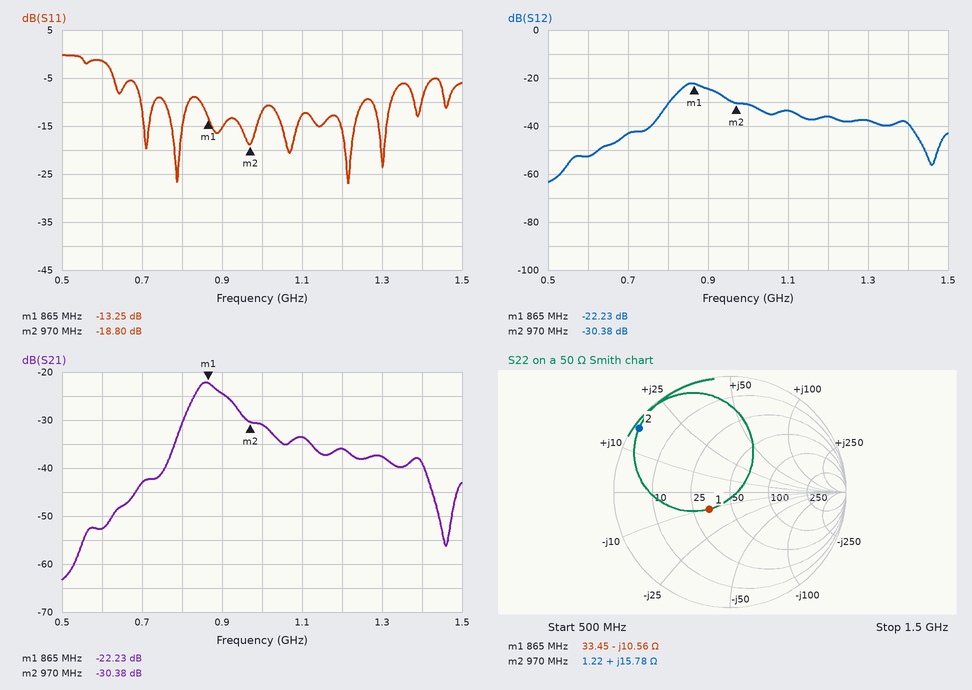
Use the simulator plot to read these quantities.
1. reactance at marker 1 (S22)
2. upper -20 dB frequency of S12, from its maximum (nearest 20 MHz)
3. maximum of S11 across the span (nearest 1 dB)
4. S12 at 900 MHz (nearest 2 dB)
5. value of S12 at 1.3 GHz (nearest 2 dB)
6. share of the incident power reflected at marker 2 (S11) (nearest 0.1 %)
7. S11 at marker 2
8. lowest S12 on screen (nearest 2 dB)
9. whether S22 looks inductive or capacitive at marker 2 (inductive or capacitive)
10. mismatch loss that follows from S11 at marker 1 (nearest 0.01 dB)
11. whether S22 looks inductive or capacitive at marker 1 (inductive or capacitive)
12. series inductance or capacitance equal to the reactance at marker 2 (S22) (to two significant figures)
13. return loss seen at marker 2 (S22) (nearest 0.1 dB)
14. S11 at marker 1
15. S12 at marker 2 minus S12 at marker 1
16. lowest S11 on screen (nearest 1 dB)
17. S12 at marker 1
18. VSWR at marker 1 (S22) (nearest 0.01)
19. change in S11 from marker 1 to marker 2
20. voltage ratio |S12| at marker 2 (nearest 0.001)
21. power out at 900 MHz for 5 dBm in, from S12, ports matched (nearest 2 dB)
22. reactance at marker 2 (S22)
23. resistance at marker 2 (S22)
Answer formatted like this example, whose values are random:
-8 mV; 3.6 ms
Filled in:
-10.56 Ω; 1.42 GHz; 0 dB; -24 dB; -38 dB; 1.3 %; -18.80 dB; -64 dB; inductive; 0.21 dB; capacitive; 2.6 nH; 0.4 dB; -13.25 dB; -8.15 dB; -27 dB; -22.23 dB; 1.61; -5.55 dB; 0.030; -20 dBm; +15.78 Ω; 1.22 Ω
